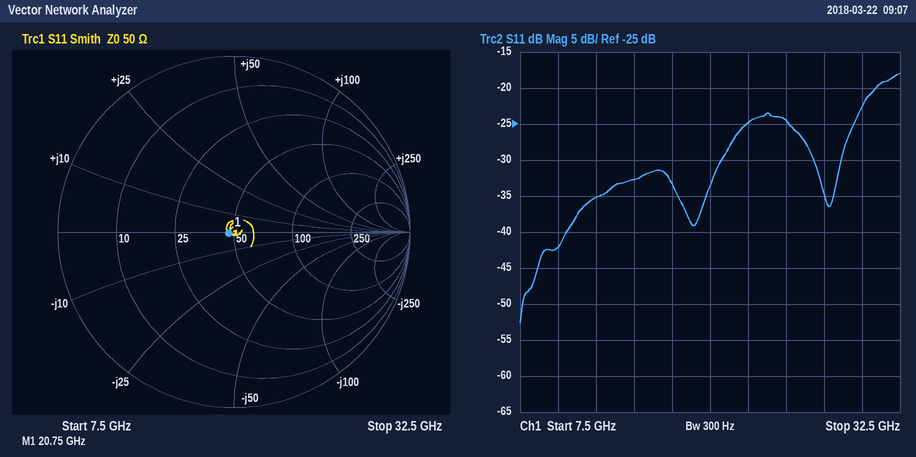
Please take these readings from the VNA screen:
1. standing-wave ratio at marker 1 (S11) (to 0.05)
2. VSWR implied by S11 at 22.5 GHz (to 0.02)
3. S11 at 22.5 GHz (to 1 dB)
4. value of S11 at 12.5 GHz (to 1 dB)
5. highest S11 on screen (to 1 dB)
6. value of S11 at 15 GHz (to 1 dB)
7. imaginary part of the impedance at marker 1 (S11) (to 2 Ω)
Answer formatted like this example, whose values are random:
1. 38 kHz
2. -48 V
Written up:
1. 1.05
2. 1.12
3. -25 dB
4. -35 dB
5. -18 dB
6. -33 dB
7. 0 Ω
